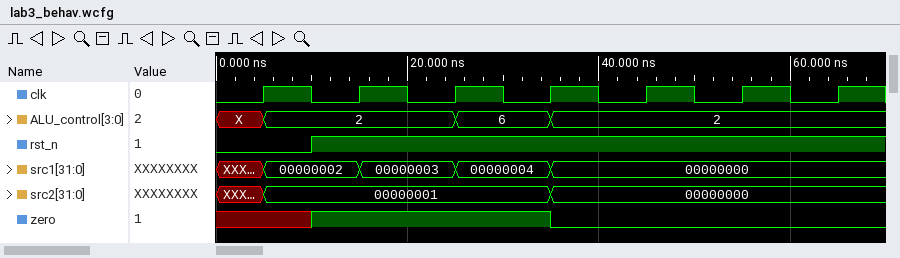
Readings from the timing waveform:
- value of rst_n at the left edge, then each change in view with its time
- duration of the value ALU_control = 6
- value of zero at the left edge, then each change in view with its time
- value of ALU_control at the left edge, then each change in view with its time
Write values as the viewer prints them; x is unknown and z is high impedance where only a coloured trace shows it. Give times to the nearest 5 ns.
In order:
0, 1 at 10 ns
10 ns
x, 1 at 10 ns, 0 at 35 ns
X, 2 at 5 ns, 6 at 25 ns, 2 at 35 ns
